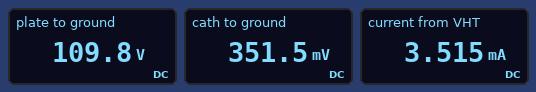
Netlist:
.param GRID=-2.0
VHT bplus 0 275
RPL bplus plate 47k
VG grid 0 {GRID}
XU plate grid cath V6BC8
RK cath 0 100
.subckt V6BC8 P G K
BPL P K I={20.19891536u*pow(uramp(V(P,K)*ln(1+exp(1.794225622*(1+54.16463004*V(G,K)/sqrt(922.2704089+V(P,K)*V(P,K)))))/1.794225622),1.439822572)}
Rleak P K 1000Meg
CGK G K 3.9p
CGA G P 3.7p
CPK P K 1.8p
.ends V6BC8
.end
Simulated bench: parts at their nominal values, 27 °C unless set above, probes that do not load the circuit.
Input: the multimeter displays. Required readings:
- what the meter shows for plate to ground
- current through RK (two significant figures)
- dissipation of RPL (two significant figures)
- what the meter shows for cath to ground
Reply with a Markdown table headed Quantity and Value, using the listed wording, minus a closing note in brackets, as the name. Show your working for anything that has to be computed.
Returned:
| Quantity | Value |
|---|---|
| what the meter shows for plate to ground | 109.8 V |
| current through RK | (351.5 mV) / 100 Ω = 3.5 mA |
| dissipation of RPL | (275 V - 109.8 V)^2 / 47 kΩ = 580 mW |
| what the meter shows for cath to ground | 351.5 mV |
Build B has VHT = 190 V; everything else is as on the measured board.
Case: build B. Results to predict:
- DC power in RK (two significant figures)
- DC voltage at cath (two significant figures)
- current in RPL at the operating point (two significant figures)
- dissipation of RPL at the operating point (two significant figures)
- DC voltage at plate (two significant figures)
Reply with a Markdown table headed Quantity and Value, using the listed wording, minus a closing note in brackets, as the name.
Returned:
| Quantity | Value |
|---|---|
| DC power in RK | 440 µW |
| DC voltage at cath | 210 mV |
| current in RPL at the operating point | 2.1 mA |
| dissipation of RPL at the operating point | 210 mW |
| DC voltage at plate | 91 V |
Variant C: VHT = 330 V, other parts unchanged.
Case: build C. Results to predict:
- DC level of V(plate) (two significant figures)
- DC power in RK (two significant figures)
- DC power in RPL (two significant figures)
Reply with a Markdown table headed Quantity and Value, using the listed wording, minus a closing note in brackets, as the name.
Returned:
| Quantity | Value |
|---|---|
| DC level of V(plate) | 120 V |
| DC power in RK | 2.0 mW |
| DC power in RPL | 930 mW |
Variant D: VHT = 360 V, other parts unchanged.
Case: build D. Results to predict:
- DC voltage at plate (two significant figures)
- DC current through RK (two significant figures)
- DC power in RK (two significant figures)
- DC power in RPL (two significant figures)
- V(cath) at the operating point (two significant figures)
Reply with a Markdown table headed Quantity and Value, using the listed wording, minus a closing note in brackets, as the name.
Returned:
| Quantity | Value |
|---|---|
| DC voltage at plate | 130 V |
| DC current through RK | 5.0 mA |
| DC power in RK | 2.5 mW |
| DC power in RPL | 1.2 W |
| V(cath) at the operating point | 500 mV |
